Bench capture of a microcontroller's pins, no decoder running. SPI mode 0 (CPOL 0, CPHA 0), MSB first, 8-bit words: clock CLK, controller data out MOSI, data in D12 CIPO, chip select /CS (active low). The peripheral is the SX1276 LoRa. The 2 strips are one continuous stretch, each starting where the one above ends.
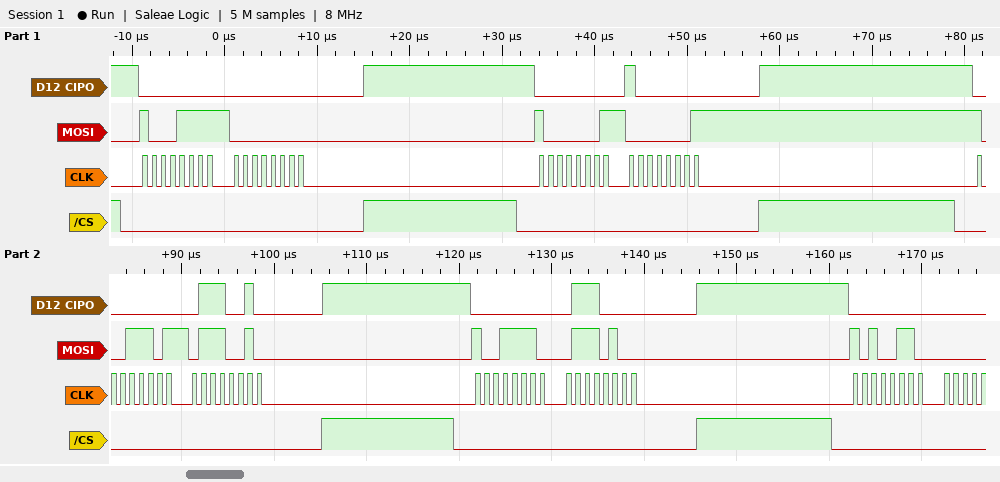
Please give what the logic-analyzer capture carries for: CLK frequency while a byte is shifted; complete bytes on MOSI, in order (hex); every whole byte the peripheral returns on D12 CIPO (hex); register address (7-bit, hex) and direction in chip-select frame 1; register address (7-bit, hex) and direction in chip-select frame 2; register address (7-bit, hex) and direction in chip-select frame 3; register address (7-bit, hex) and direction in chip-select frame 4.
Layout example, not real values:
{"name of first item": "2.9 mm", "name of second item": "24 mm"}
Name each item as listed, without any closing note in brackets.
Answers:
{"CLK frequency while a byte is shifted": "1 MHz", "complete bytes on MOSI, in order": "8F 00 81 01 9D 72 9E 74 A6", "every whole byte the peripheral returns on D12 CIPO": "00 00 00 80 00 72 00 70 00", "register address (7-bit, hex) and direction in chip-select frame 1": "0x0F write", "register address (7-bit, hex) and direction in chip-select frame 2": "0x01 write", "register address (7-bit, hex) and direction in chip-select frame 3": "0x1D write", "register address (7-bit, hex) and direction in chip-select frame 4": "0x1E write"}
